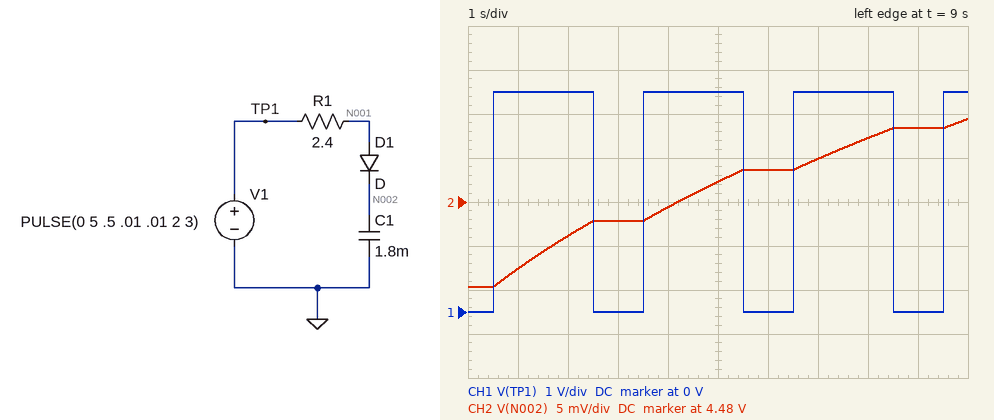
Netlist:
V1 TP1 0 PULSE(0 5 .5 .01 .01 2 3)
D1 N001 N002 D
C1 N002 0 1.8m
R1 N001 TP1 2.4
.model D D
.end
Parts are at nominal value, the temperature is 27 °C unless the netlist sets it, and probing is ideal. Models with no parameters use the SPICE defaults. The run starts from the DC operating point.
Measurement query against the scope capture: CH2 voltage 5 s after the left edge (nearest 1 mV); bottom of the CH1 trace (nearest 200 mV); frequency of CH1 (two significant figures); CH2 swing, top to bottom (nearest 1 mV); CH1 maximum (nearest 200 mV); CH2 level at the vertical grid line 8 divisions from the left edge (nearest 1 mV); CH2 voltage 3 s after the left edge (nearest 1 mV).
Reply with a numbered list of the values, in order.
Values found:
1. 4.482 V
2. 0 V
3. 330 mHz
4. 19 mV
5. 5.0 V
6. 4.487 V
7. 4.478 V
